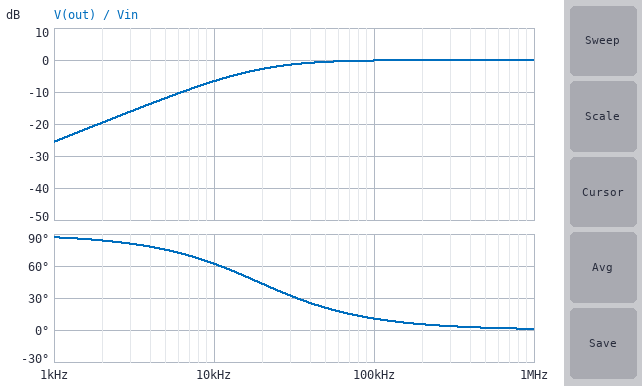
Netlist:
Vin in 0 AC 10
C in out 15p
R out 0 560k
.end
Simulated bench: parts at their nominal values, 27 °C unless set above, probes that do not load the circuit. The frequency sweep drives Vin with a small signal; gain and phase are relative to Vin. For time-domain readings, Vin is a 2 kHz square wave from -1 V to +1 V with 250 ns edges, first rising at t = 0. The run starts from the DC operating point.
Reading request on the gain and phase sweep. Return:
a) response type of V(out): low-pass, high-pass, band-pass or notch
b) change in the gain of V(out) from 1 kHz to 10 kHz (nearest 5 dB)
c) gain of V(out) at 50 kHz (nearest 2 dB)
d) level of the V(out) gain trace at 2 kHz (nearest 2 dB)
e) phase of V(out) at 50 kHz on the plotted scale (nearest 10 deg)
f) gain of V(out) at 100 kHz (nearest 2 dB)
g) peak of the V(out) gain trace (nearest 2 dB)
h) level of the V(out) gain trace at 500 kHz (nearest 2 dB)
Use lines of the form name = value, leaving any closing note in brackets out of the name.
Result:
response type of V(out): low-pass, high-pass, band-pass or notch = high-pass
change in the gain of V(out) from 1 kHz to 10 kHz = 20 dB
gain of V(out) at 50 kHz = 0 dB
level of the V(out) gain trace at 2 kHz = -20 dB
phase of V(out) at 50 kHz on the plotted scale = 20 deg
gain of V(out) at 100 kHz = 0 dB
peak of the V(out) gain trace = 0 dB
level of the V(out) gain trace at 500 kHz = 0 dB
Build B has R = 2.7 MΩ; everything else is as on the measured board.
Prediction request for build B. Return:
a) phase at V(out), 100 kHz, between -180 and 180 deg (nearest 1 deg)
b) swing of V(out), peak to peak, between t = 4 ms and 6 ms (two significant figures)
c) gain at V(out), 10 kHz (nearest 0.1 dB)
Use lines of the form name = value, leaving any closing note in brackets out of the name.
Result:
phase at V(out), 100 kHz, between -180 and 180 deg = 2 deg
swing of V(out), peak to peak, between t = 4 ms and 6 ms = 4.0 V
gain at V(out), 10 kHz = -0.6 dB
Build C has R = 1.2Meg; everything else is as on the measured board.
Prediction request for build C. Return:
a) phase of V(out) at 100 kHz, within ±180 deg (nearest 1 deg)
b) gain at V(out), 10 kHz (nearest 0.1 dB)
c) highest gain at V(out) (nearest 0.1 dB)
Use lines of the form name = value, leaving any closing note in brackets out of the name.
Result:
phase of V(out) at 100 kHz, within ±180 deg = 5 deg
gain at V(out), 10 kHz = -2.5 dB
highest gain at V(out) = 0 dB
